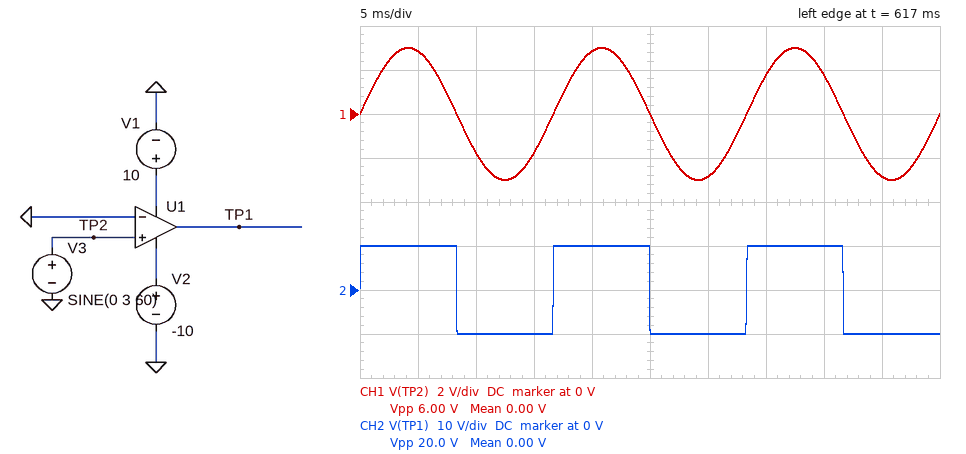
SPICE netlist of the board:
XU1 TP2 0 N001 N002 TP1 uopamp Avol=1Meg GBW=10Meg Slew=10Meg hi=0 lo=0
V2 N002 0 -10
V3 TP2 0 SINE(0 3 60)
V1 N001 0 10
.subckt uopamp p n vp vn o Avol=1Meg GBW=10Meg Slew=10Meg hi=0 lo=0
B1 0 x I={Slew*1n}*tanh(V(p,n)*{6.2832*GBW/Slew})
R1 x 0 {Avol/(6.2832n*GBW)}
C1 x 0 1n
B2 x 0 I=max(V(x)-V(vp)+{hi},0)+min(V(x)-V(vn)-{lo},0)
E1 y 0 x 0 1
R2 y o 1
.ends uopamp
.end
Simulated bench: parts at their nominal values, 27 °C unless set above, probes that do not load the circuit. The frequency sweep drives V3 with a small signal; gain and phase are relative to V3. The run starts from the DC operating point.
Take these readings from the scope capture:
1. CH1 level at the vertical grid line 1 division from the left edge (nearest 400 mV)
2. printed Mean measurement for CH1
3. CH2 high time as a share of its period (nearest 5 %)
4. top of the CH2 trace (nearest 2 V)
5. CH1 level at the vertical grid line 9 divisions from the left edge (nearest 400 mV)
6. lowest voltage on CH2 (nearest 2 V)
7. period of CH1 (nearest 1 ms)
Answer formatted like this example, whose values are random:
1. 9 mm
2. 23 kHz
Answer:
1. 2.8 V
2. 0.00 V
3. 50 %
4. 10 V
5. -2.8 V
6. -10 V
7. 17 ms
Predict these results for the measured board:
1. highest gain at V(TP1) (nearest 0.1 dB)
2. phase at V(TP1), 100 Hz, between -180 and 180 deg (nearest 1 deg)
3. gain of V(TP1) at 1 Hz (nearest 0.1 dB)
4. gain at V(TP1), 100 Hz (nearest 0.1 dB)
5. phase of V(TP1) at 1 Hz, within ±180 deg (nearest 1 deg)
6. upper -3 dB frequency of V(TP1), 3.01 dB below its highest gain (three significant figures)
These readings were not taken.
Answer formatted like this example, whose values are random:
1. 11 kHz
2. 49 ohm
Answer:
1. 120.0 dB
2. -84 deg
3. 120.0 dB
4. 100.0 dB
5. -6 deg
6. 10.0 Hz
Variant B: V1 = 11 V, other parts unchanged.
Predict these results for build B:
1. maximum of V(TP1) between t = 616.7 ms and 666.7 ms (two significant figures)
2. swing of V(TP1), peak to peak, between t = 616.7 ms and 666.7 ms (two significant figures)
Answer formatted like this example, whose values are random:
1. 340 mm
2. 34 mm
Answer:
1. 11 V
2. 21 V
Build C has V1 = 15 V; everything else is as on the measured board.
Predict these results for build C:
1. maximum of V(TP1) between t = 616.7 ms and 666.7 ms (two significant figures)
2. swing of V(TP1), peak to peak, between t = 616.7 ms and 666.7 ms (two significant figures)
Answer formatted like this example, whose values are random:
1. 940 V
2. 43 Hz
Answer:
1. 15 V
2. 25 V
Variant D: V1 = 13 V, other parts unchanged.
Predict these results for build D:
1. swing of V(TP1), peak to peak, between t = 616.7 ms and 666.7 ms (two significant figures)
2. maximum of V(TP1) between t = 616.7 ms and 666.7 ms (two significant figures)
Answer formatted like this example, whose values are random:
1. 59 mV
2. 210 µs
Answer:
1. 23 V
2. 13 V
